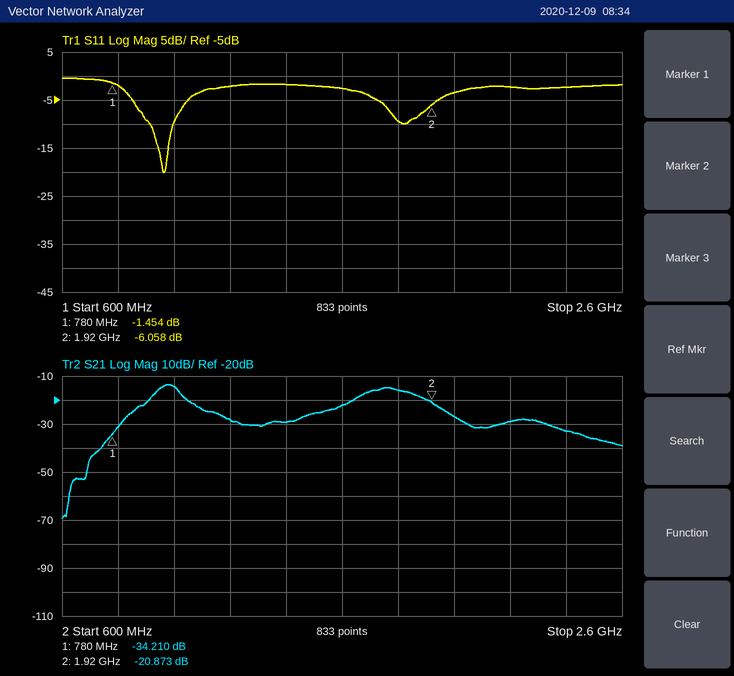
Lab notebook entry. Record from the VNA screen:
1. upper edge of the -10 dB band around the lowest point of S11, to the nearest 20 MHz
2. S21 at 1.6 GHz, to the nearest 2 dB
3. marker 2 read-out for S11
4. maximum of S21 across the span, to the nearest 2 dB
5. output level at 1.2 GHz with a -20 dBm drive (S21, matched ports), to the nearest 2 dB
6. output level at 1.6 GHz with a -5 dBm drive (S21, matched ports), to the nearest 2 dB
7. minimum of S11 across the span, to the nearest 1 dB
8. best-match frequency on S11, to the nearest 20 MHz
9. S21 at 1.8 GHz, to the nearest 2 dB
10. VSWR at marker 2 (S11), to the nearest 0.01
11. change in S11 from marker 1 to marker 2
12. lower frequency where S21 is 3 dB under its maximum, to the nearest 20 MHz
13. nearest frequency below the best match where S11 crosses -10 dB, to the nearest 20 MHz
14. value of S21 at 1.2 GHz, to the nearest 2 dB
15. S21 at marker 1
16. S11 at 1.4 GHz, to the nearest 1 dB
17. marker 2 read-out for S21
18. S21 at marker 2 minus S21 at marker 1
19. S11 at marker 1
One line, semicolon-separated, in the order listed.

1.00 GHz; -22 dB; -6.058 dB; -14 dB; -48 dBm; -28 dBm; -20 dB; 960 MHz; -16 dB; 2.98; -4.604 dB; 940 MHz; 920 MHz; -28 dB; -34.210 dB; -2 dB; -20.873 dB; 13.337 dB; -1.454 dB
